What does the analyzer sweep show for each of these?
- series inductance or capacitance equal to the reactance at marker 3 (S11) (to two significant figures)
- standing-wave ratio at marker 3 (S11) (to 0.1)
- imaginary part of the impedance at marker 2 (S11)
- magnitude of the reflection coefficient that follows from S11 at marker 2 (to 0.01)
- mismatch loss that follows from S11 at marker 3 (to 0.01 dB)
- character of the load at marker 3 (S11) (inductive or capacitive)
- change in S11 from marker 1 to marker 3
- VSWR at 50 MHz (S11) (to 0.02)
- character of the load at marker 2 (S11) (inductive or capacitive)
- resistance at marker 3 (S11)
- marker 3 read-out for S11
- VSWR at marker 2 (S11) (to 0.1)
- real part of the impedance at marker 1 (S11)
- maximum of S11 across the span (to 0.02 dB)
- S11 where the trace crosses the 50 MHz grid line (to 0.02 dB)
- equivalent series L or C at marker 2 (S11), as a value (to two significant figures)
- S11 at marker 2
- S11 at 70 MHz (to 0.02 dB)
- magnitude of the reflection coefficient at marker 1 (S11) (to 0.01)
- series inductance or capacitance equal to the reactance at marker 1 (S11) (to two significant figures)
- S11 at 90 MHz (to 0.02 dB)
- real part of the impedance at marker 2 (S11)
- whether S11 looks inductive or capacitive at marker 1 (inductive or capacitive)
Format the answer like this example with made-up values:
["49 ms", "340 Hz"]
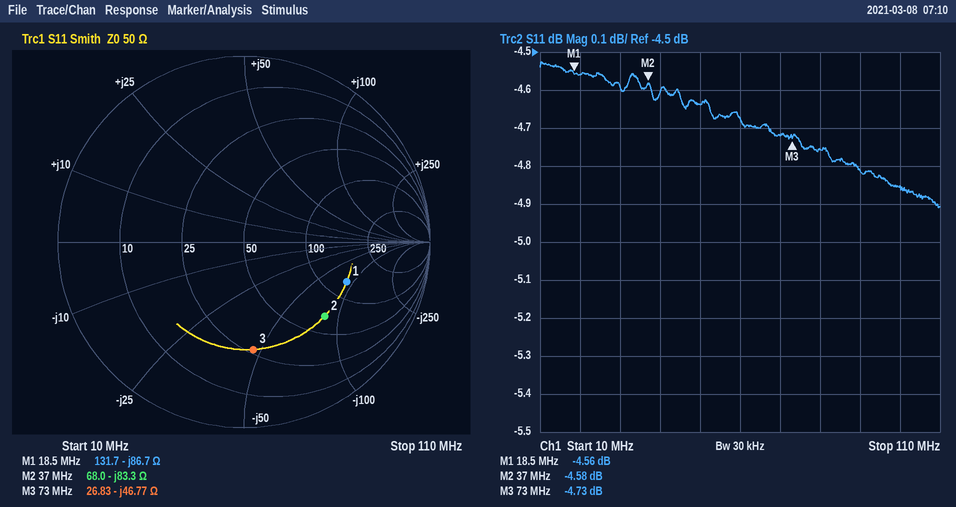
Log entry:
["47 pF", "3.8", "-83.3 Ω", "0.59", "1.78 dB", "capacitive", "-0.17 dB", "3.84", "capacitive", "26.83 Ω", "-4.73 dB", "3.9", "131.7 Ω", "-4.52 dB", "-4.64 dB", "52 pF", "-4.58 dB", "-4.72 dB", "0.59", "99 pF", "-4.82 dB", "68.0 Ω", "capacitive"]
